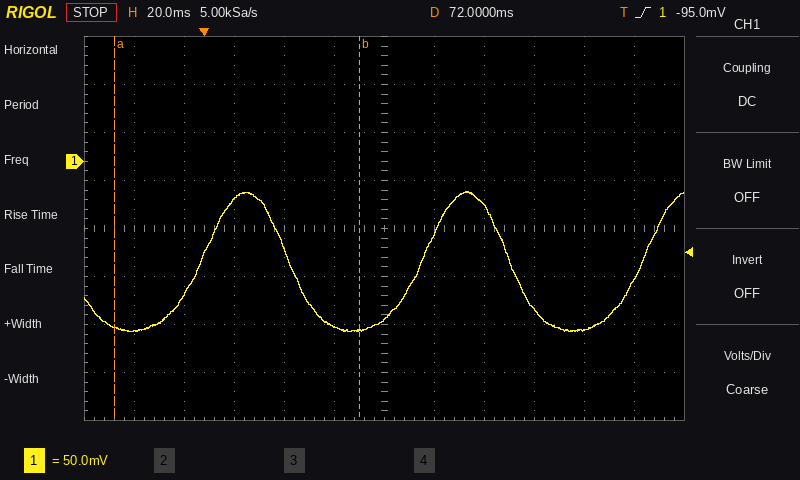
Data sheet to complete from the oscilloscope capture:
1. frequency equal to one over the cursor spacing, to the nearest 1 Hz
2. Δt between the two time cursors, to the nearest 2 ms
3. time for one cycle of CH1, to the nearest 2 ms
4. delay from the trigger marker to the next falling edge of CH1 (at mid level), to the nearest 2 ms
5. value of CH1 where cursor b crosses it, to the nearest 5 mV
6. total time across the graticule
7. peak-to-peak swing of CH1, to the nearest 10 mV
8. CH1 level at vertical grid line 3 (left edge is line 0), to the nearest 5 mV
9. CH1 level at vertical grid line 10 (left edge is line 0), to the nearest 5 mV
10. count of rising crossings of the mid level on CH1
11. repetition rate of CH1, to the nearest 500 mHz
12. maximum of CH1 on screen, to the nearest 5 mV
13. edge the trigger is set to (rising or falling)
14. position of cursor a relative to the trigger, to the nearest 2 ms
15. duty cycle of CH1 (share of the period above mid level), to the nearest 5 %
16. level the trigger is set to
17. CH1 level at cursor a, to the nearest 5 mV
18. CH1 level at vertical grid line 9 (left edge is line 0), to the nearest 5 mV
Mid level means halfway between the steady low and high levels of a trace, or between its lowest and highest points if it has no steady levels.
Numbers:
10 Hz
98 ms
88 ms
34 ms
-175 mV
240 ms
150 mV
-40 mV
-175 mV
3
11.5 Hz
-30 mV
rising
-36 ms
40 %
-95.0 mV
-175 mV
-155 mV
